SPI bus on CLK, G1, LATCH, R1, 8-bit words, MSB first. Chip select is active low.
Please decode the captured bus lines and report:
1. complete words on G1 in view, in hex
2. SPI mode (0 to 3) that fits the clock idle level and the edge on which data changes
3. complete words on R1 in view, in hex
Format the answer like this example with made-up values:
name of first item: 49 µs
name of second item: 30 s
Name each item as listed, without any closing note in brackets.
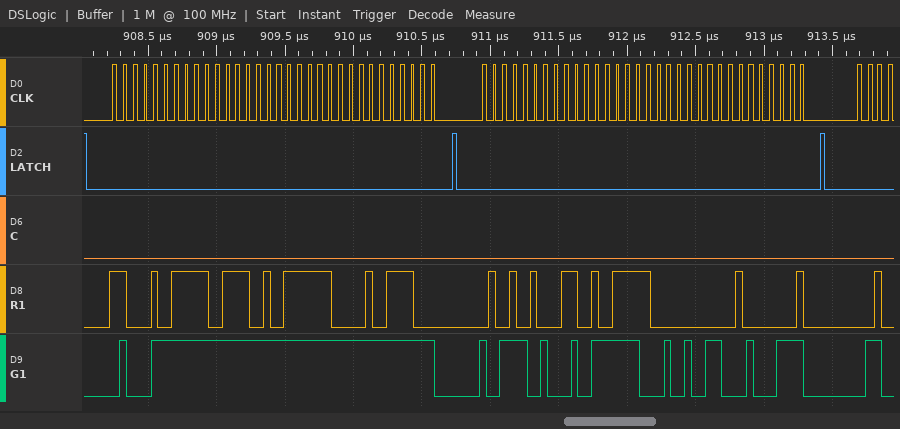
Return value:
complete words on G1 in view, in hex: 4F, FF, FF, FF, BA, 5F, 2B, 27
SPI mode (0 to 3) that fits the clock idle level and the edge on which data changes: 0
complete words on R1 in view, in hex: CB, DD, 7C, 5C, 54, D7, 80, 41
